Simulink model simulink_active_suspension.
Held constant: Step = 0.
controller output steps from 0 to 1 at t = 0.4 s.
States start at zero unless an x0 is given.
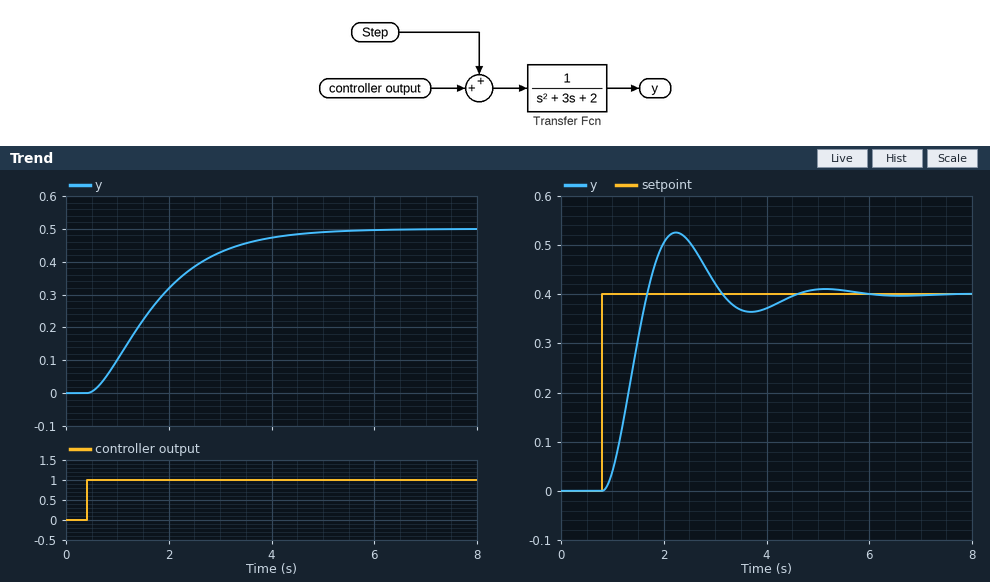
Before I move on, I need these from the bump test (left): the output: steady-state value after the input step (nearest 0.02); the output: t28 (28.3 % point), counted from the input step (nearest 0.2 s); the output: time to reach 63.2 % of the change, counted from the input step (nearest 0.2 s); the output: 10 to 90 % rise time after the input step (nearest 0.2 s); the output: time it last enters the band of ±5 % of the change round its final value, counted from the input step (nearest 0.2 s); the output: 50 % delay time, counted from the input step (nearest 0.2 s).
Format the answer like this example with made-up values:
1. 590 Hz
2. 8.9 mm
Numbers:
1. 0.50
2. 0.8 s
3. 1.6 s
4. 2.6 s
5. 3.6 s
6. 1.2 s
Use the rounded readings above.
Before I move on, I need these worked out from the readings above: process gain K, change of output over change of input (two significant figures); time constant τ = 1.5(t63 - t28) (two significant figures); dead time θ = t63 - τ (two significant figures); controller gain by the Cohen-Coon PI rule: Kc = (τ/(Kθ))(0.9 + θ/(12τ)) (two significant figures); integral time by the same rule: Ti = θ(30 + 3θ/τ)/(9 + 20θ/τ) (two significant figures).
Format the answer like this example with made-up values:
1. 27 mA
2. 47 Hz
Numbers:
1. 0.50
2. 1.2 s
3. 0.40 s
4. 5.6
5. 0.79 s
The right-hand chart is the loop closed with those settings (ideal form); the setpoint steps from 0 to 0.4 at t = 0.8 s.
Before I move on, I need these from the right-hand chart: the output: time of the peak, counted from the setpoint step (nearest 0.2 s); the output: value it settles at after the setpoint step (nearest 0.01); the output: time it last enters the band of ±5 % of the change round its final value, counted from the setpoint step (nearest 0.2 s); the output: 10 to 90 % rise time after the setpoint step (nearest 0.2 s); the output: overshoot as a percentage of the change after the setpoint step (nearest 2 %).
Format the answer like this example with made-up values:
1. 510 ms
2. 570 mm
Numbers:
1. 1.4 s
2. 0.40
3. 3.4 s
4. 0.6 s
5. 32 %
